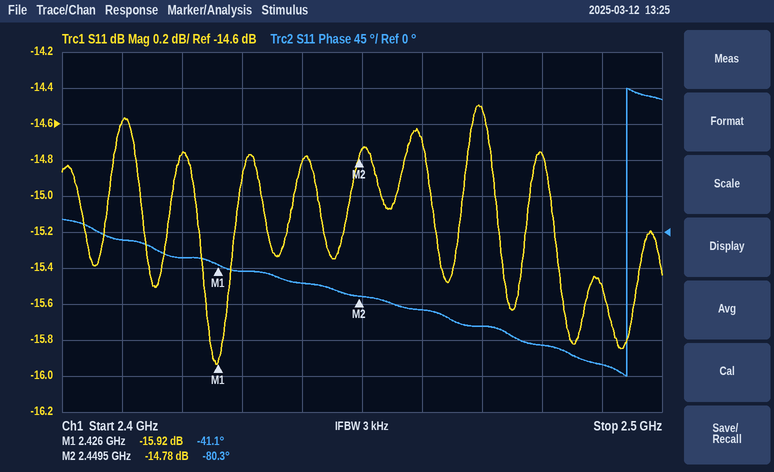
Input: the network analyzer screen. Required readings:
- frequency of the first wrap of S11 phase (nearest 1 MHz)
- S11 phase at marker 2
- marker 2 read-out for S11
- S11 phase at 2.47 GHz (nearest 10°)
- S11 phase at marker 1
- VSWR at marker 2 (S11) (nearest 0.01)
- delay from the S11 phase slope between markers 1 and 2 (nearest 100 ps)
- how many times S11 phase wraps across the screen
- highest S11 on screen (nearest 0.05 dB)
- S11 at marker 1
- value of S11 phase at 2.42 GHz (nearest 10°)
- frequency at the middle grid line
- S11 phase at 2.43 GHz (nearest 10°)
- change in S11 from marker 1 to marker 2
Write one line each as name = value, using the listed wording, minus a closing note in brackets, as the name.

frequency of the first wrap of S11 phase = 2.494 GHz
S11 phase at marker 2 = -80.3°
marker 2 read-out for S11 = -14.78 dB
S11 phase at 2.47 GHz = -120°
S11 phase at marker 1 = -41.1°
VSWR at marker 2 (S11) = 1.45
delay from the S11 phase slope between markers 1 and 2 = 4.6 ns
how many times S11 phase wraps across the screen = 1
highest S11 on screen = -14.50 dB
S11 at marker 1 = -15.92 dB
value of S11 phase at 2.42 GHz = -30°
frequency at the middle grid line = 2.45 GHz
S11 phase at 2.43 GHz = -50°
change in S11 from marker 1 to marker 2 = 1.14 dB
